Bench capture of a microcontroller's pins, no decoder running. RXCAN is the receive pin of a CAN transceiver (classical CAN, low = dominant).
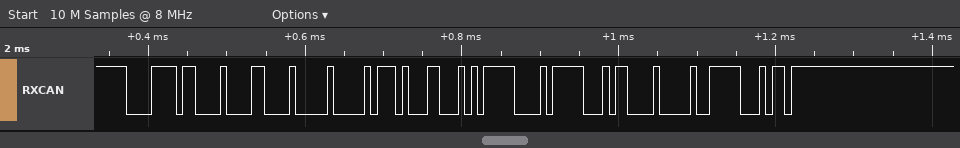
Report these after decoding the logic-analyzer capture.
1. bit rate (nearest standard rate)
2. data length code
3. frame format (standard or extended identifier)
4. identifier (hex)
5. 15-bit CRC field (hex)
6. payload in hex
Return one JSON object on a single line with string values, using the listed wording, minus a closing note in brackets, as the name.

{"bit rate": "125 kbit/s", "data length code": "8", "frame format": "standard", "identifier": "0x0F6", "15-bit CRC field": "0x03E5", "payload in hex": "61 00 1D 18 AF 8B E5 84"}
